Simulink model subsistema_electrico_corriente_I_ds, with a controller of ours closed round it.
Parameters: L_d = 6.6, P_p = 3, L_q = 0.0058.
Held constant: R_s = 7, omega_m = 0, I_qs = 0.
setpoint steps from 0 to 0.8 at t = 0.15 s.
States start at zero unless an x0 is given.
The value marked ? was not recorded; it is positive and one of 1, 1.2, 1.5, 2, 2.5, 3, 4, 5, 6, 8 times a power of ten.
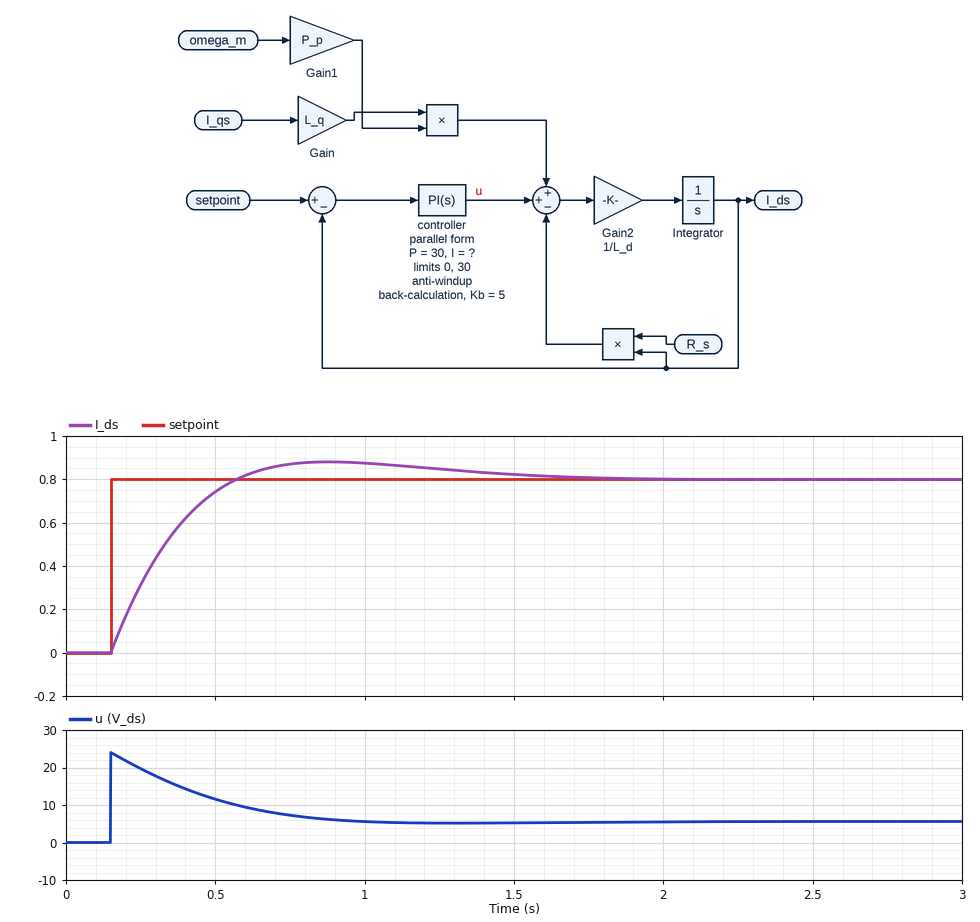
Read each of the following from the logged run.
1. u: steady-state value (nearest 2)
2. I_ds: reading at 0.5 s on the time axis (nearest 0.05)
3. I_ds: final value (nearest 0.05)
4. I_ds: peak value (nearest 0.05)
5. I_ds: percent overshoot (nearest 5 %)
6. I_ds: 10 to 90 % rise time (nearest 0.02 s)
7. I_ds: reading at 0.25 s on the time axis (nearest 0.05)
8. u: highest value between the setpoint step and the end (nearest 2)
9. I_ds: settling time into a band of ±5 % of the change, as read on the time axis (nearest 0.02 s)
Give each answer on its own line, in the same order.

6
0.75
0.80
0.90
10 %
0.30 s
0.30
24
1.32 s
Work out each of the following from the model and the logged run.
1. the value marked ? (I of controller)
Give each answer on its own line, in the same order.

80
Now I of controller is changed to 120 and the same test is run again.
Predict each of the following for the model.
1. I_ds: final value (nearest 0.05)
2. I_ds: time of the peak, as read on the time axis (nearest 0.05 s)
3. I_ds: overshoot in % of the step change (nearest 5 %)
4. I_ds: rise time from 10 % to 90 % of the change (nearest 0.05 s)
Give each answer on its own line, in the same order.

0.80
0.75 s
15 %
0.25 s
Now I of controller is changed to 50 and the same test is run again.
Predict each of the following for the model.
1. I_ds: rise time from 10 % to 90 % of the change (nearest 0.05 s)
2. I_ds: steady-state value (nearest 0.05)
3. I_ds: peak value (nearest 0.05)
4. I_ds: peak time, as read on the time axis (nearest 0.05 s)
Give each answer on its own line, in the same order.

0.40 s
0.80
0.85
1.10 s
